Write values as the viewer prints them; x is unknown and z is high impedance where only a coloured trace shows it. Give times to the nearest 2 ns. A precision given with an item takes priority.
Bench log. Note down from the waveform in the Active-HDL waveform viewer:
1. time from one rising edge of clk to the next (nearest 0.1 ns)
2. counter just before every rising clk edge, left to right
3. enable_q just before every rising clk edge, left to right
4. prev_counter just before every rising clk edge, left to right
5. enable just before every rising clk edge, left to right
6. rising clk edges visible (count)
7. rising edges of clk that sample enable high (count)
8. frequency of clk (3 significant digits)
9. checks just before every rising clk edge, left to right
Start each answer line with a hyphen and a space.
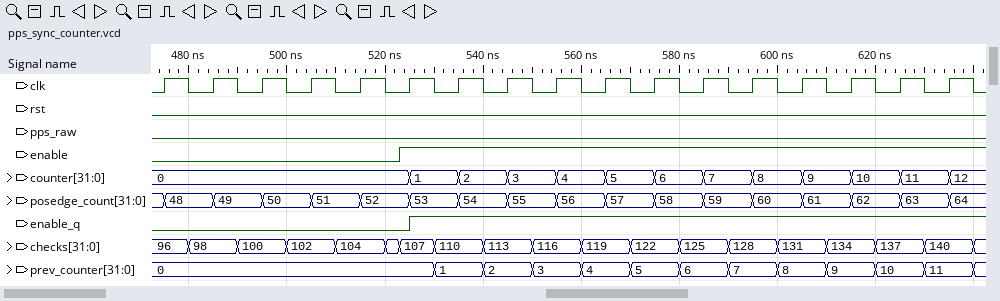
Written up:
- 10 ns
- 0, 0, 0, 0, 0, 0, 1, 2, 3, 4, 5, 6, 7, 8, 9, 10, 11
- 0 0 0 0 0 0 1 1 1 1 1 1 1 1 1 1 1
- 0, 0, 0, 0, 0, 0, 1, 2, 3, 4, 5, 6, 7, 8, 9, 10, 11
- 0 0 0 0 0 1 1 1 1 1 1 1 1 1 1 1 1
- 17
- 12
- 100 MHz
- 96, 98, 100, 102, 104, 107, 110, 113, 116, 119, 122, 125, 128, 131, 134, 137, 140
